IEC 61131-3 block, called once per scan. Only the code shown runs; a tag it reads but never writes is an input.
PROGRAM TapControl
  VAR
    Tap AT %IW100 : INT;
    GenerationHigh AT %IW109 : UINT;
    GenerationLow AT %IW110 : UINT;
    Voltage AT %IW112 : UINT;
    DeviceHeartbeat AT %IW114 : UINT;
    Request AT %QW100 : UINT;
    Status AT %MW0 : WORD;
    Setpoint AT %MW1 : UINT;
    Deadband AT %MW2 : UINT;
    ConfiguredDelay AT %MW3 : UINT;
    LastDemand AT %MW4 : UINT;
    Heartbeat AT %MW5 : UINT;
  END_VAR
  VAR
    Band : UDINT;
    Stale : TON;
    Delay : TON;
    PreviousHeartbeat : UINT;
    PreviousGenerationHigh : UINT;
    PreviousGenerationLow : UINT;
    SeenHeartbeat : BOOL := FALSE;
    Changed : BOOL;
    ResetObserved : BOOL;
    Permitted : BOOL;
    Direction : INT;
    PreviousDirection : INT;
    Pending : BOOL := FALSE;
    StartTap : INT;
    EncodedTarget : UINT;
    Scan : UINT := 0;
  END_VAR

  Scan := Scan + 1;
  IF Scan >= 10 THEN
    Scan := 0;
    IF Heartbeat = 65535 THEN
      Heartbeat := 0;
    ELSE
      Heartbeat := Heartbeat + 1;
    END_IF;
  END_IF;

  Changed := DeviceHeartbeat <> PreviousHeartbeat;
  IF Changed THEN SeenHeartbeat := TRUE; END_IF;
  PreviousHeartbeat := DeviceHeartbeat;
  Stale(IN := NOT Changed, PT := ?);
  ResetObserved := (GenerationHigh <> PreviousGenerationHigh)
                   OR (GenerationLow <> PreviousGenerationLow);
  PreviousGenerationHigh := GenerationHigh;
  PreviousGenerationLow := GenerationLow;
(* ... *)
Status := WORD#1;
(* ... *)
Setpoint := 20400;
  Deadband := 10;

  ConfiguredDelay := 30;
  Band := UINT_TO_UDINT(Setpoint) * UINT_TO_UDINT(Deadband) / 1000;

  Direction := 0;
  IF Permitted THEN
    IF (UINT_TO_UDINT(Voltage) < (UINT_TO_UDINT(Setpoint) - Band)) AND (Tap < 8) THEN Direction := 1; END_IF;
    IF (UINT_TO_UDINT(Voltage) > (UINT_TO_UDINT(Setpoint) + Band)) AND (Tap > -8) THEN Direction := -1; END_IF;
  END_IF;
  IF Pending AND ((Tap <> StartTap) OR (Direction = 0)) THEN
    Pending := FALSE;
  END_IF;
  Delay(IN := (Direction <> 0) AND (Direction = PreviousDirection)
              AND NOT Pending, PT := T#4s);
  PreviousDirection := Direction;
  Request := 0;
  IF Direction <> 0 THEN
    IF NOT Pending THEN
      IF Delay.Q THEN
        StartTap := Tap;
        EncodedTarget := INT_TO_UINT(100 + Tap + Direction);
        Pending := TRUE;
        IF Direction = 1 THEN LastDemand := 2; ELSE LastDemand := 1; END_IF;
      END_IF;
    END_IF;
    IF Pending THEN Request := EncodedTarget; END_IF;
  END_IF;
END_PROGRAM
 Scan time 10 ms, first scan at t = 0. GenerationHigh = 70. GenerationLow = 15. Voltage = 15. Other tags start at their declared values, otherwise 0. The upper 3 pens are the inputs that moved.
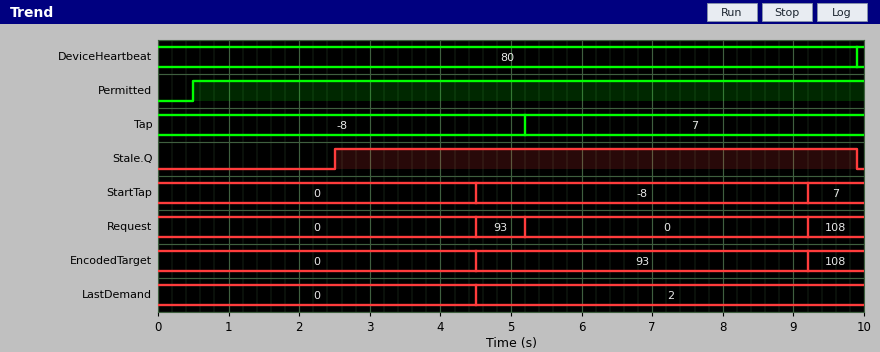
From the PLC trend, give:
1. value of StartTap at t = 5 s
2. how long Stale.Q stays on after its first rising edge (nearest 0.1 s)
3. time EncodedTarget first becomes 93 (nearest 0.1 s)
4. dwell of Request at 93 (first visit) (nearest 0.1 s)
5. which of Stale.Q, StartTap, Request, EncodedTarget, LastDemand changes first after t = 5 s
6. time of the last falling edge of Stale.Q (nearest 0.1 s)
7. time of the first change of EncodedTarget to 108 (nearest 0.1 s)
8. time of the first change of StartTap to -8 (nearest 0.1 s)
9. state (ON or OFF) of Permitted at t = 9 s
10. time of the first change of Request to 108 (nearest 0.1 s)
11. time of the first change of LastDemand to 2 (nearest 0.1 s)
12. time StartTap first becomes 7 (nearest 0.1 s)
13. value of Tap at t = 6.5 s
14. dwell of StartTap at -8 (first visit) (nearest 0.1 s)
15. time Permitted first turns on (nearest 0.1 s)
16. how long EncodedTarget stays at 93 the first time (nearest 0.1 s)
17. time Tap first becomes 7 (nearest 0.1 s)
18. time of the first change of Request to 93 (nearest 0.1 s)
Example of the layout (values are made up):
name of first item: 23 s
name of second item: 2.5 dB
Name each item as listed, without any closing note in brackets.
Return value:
value of StartTap at t = 5 s: -8
how long Stale.Q stays on after its first rising edge: 7.4 s
time EncodedTarget first becomes 93: 4.5 s
dwell of Request at 93 (first visit): 0.7 s
which of Stale.Q, StartTap, Request, EncodedTarget, LastDemand changes first after t = 5 s: Request
time of the last falling edge of Stale.Q: 9.9 s
time of the first change of EncodedTarget to 108: 9.2 s
time of the first change of StartTap to -8: 4.5 s
state (ON or OFF) of Permitted at t = 9 s: ON
time of the first change of Request to 108: 9.2 s
time of the first change of LastDemand to 2: 4.5 s
time StartTap first becomes 7: 9.2 s
value of Tap at t = 6.5 s: 7
dwell of StartTap at -8 (first visit): 4.7 s
time Permitted first turns on: 0.5 s
how long EncodedTarget stays at 93 the first time: 4.7 s
time Tap first becomes 7: 5.2 s
time of the first change of Request to 93: 4.5 s
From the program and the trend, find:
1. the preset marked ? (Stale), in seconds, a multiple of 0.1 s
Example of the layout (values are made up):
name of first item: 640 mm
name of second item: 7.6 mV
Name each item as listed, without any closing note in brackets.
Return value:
the preset marked ? (Stale), in seconds, a multiple of 0.1 s: 2.5 s
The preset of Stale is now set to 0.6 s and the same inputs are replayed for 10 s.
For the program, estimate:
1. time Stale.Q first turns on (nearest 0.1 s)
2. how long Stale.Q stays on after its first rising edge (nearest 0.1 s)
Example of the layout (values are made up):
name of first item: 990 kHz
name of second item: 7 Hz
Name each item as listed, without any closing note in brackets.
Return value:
time Stale.Q first turns on: 0.6 s
how long Stale.Q stays on after its first rising edge: 9.3 s
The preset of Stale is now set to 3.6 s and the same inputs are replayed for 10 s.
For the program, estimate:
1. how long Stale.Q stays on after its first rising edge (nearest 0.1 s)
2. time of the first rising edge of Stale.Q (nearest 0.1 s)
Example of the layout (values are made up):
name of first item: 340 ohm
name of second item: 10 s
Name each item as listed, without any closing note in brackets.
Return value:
how long Stale.Q stays on after its first rising edge: 6.3 s
time of the first rising edge of Stale.Q: 3.6 s
